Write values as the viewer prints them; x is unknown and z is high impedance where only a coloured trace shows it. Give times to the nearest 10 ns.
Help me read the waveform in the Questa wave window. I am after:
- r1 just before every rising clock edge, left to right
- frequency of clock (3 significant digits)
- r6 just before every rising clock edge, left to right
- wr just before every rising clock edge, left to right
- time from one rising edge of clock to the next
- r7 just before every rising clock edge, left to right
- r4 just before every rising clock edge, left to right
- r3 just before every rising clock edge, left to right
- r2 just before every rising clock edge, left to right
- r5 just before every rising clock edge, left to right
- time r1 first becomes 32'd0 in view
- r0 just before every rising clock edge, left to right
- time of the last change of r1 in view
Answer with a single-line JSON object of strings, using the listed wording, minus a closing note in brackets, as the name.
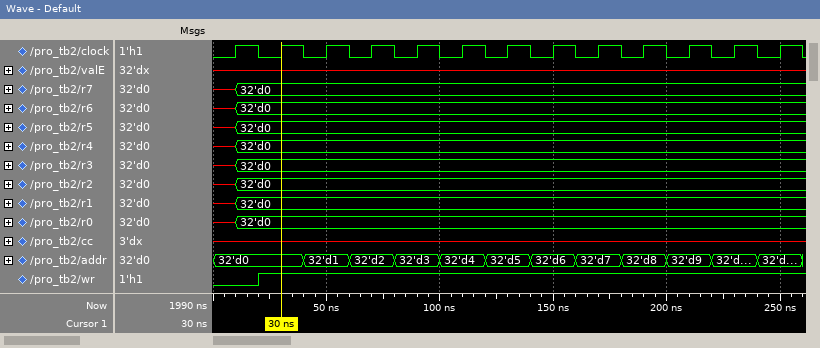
{"r1 just before every rising clock edge, left to right": "x, 32'd0, 32'd0, 32'd0, 32'd0, 32'd0, 32'd0, 32'd0, 32'd0, 32'd0, 32'd0, 32'd0, 32'd0", "frequency of clock": "50.0 MHz", "r6 just before every rising clock edge, left to right": "x, 32'd0, 32'd0, 32'd0, 32'd0, 32'd0, 32'd0, 32'd0, 32'd0, 32'd0, 32'd0, 32'd0, 32'd0", "wr just before every rising clock edge, left to right": "0 1 1 1 1 1 1 1 1 1 1 1 1", "time from one rising edge of clock to the next": "20 ns", "r7 just before every rising clock edge, left to right": "x, 32'd0, 32'd0, 32'd0, 32'd0, 32'd0, 32'd0, 32'd0, 32'd0, 32'd0, 32'd0, 32'd0, 32'd0", "r4 just before every rising clock edge, left to right": "x, 32'd0, 32'd0, 32'd0, 32'd0, 32'd0, 32'd0, 32'd0, 32'd0, 32'd0, 32'd0, 32'd0, 32'd0", "r3 just before every rising clock edge, left to right": "x, 32'd0, 32'd0, 32'd0, 32'd0, 32'd0, 32'd0, 32'd0, 32'd0, 32'd0, 32'd0, 32'd0, 32'd0", "r2 just before every rising clock edge, left to right": "x, 32'd0, 32'd0, 32'd0, 32'd0, 32'd0, 32'd0, 32'd0, 32'd0, 32'd0, 32'd0, 32'd0, 32'd0", "r5 just before every rising clock edge, left to right": "x, 32'd0, 32'd0, 32'd0, 32'd0, 32'd0, 32'd0, 32'd0, 32'd0, 32'd0, 32'd0, 32'd0, 32'd0", "time r1 first becomes 32'd0 in view": "10 ns", "r0 just before every rising clock edge, left to right": "x, 32'd0, 32'd0, 32'd0, 32'd0, 32'd0, 32'd0, 32'd0, 32'd0, 32'd0, 32'd0, 32'd0, 32'd0", "time of the last change of r1 in view": "10 ns"}
